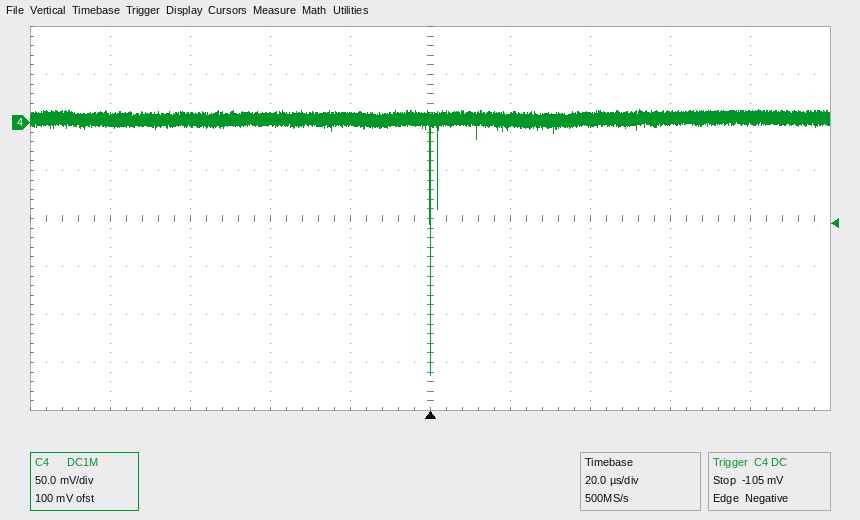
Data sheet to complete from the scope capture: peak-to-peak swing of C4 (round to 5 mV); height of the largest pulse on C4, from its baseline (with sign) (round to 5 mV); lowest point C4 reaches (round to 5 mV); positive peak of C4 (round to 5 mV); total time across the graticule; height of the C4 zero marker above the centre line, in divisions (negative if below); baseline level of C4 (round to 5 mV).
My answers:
275 mV
-265 mV
-260 mV
15 mV
200 µs
+2.0 div
5 mV
